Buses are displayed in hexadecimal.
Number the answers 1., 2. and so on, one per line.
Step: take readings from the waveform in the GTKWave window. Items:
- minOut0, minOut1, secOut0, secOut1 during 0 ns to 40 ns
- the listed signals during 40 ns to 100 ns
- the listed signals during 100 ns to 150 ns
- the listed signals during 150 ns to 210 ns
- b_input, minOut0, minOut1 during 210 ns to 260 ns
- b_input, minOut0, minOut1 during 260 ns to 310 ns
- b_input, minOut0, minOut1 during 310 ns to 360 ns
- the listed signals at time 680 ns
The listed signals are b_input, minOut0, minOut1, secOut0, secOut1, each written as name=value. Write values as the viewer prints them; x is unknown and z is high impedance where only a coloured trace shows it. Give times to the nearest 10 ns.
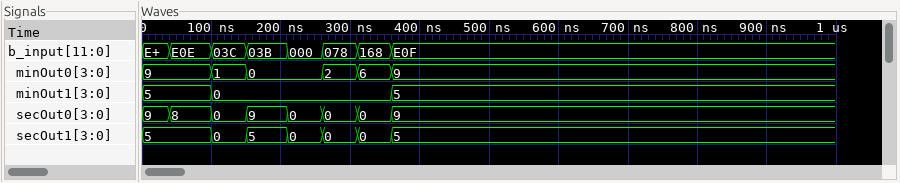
1. minOut0=9, minOut1=5, secOut0=9, secOut1=5
2. b_input=E0E, minOut0=9, minOut1=5, secOut0=8, secOut1=5
3. b_input=03C, minOut0=1, minOut1=0, secOut0=0, secOut1=0
4. b_input=03B, minOut0=0, minOut1=0, secOut0=9, secOut1=5
5. b_input=000, minOut0=0, minOut1=0
6. b_input=078, minOut0=2, minOut1=0
7. b_input=168, minOut0=6, minOut1=0
8. b_input=E0F, minOut0=9, minOut1=5, secOut0=9, secOut1=5
